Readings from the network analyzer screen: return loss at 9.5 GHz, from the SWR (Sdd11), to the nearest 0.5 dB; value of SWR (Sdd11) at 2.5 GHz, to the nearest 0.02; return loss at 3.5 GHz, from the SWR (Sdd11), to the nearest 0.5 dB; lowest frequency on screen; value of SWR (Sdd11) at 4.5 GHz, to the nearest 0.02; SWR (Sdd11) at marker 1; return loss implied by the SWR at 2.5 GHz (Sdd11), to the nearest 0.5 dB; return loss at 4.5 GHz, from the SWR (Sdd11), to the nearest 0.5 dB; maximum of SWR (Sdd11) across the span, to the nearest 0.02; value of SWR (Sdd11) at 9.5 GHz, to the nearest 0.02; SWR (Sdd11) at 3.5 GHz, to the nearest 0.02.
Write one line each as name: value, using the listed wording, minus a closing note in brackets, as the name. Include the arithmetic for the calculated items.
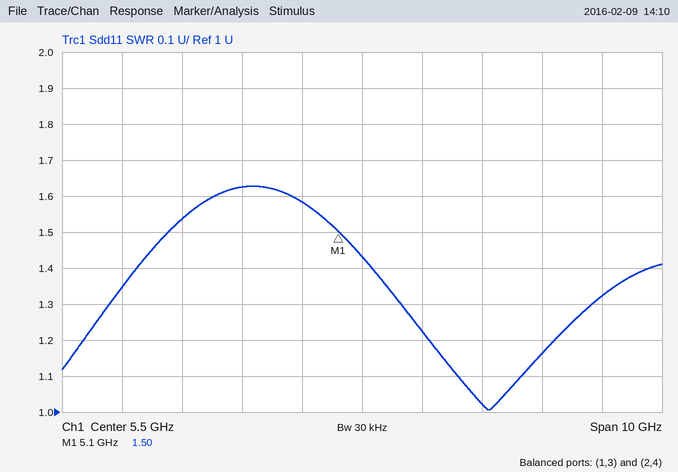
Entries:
return loss at 9.5 GHz, from the SWR (Sdd11), to the nearest 0.5 dB: −20 log10((1.32 − 1)/(1.32 + 1)) ≈ 17.2 dB, so 17.0 dB to the nearest 0.5 dB
value of SWR (Sdd11) at 2.5 GHz, to the nearest 0.02: 1.54
return loss at 3.5 GHz, from the SWR (Sdd11), to the nearest 0.5 dB: −20 log10((1.62 − 1)/(1.62 + 1)) ≈ 12.5 dB
lowest frequency on screen: 500 MHz
value of SWR (Sdd11) at 4.5 GHz, to the nearest 0.02: 1.58
SWR (Sdd11) at marker 1: 1.50
return loss implied by the SWR at 2.5 GHz (Sdd11), to the nearest 0.5 dB: −20 log10((1.54 − 1)/(1.54 + 1)) ≈ 13.4 dB, so 13.5 dB to the nearest 0.5 dB
return loss at 4.5 GHz, from the SWR (Sdd11), to the nearest 0.5 dB: −20 log10((1.58 − 1)/(1.58 + 1)) ≈ 13.0 dB
maximum of SWR (Sdd11) across the span, to the nearest 0.02: 1.62
value of SWR (Sdd11) at 9.5 GHz, to the nearest 0.02: 1.32
SWR (Sdd11) at 3.5 GHz, to the nearest 0.02: 1.62
